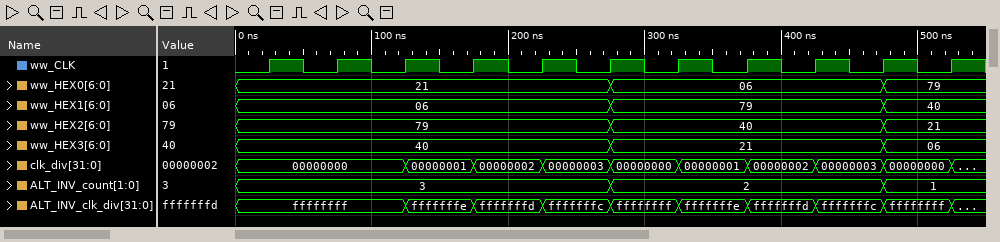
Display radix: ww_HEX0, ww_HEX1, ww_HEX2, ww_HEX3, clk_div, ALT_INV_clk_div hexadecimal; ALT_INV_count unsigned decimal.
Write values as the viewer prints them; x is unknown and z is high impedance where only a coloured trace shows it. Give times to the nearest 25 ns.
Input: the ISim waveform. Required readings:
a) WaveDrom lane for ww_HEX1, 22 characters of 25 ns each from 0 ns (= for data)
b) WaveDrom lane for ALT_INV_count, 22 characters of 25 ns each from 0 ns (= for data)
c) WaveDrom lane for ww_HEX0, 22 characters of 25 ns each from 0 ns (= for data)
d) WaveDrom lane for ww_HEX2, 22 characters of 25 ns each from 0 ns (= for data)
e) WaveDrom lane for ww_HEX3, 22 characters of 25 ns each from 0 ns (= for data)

{name: 'ww_HEX1', wave: '=..........=.......=..', data: '06 79 40'}
{name: 'ALT_INV_count', wave: '=..........=.......=..', data: '3 2 1'}
{name: 'ww_HEX0', wave: '=..........=.......=..', data: '21 06 79'}
{name: 'ww_HEX2', wave: '=..........=.......=..', data: '79 40 21'}
{name: 'ww_HEX3', wave: '=..........=.......=..', data: '40 21 06'}
